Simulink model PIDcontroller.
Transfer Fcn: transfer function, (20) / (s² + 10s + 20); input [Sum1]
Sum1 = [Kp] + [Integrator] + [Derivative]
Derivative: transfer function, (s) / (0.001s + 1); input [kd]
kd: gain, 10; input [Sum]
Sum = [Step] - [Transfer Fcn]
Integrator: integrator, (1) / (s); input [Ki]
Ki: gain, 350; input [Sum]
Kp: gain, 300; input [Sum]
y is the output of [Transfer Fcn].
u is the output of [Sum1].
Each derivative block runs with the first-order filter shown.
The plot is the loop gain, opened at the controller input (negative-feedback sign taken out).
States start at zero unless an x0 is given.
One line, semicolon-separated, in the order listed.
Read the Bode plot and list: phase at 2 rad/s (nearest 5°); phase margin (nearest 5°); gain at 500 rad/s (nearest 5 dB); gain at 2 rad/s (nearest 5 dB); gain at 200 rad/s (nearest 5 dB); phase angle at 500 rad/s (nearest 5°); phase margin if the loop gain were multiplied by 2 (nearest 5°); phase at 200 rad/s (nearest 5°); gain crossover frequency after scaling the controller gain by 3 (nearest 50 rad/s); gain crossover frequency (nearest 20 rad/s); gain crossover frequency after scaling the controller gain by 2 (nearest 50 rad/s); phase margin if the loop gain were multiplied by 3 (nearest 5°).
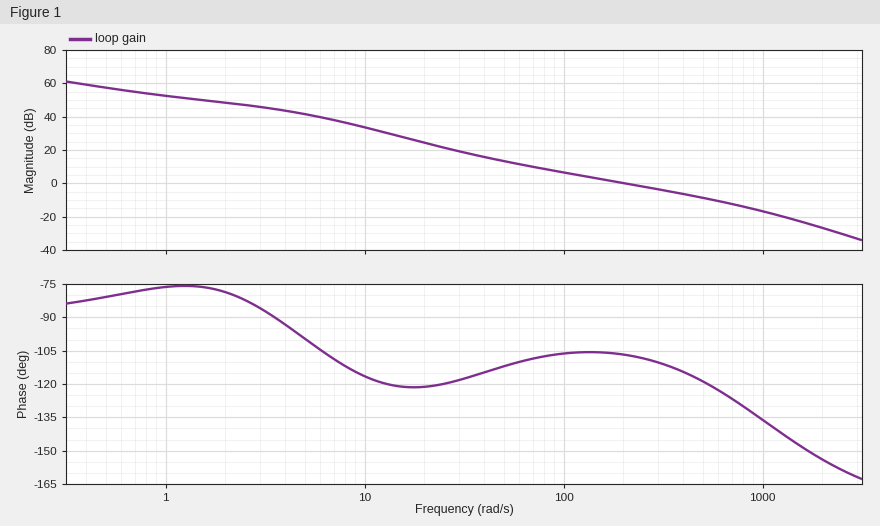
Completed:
-80°; 75°; -10 dB; 50 dB; 0 dB; -120°; 65°; -105°; 550 rad/s; 200 rad/s; 400 rad/s; 60°
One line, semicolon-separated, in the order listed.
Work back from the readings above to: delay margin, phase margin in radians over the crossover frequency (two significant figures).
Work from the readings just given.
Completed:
0.0065 s
